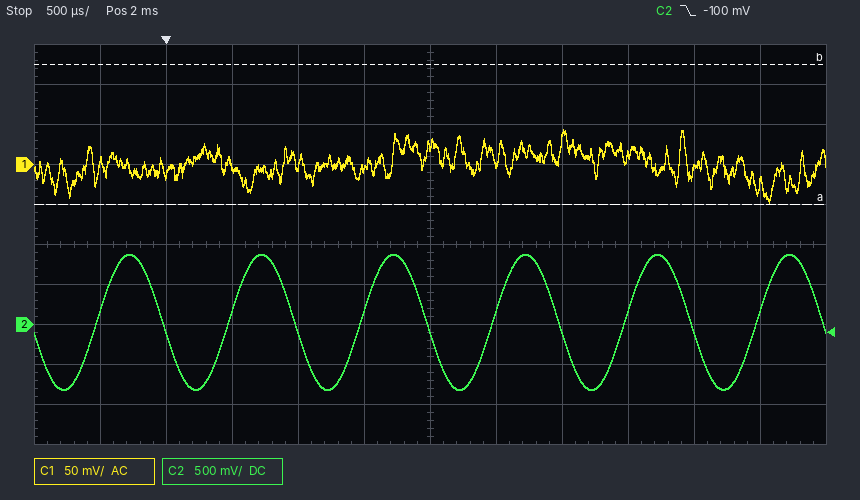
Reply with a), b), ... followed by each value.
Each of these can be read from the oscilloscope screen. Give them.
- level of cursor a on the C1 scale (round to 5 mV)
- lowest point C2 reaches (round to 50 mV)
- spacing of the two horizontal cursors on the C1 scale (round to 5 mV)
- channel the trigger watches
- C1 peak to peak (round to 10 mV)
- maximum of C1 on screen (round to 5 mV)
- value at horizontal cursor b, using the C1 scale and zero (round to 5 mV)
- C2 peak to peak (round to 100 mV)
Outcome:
a) -50 mV
b) -800 mV
c) 175 mV
d) C2
e) 90 mV
f) 45 mV
g) 125 mV
h) 1.70 V
